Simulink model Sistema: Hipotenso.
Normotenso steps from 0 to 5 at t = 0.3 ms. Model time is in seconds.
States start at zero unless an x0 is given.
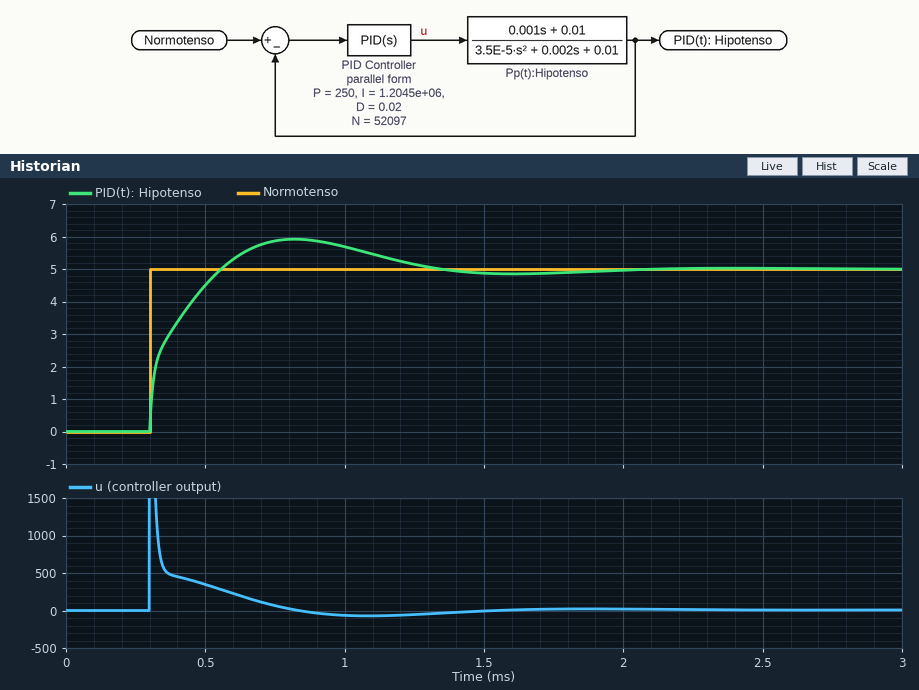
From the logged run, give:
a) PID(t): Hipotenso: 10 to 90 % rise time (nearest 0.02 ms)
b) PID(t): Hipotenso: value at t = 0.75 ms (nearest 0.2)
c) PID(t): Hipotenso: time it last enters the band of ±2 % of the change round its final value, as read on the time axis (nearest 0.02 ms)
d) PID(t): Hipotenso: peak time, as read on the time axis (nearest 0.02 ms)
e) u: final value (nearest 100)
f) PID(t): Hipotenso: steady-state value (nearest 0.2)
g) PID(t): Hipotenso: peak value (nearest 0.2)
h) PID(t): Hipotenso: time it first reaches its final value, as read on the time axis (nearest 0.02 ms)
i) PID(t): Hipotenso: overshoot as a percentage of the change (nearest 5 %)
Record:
0.20 ms
5.8
1.82 ms
0.82 ms
0
5.0
6.0
0.56 ms
20 %
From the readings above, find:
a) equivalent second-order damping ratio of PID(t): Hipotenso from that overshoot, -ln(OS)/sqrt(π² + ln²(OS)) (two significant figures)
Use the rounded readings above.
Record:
0.46
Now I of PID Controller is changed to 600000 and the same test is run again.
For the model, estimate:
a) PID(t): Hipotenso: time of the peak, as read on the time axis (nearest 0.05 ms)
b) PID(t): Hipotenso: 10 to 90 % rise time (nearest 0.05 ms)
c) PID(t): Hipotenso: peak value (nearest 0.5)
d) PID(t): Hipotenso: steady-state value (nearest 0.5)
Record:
1.00 ms
0.25 ms
5.5
5.0
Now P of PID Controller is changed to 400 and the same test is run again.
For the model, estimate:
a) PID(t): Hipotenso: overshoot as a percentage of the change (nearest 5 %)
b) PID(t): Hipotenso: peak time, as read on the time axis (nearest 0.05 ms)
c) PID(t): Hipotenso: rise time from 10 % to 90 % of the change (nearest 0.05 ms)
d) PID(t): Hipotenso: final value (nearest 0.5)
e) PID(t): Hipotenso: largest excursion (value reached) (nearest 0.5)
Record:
10 %
0.75 ms
0.15 ms
5.0
5.5
